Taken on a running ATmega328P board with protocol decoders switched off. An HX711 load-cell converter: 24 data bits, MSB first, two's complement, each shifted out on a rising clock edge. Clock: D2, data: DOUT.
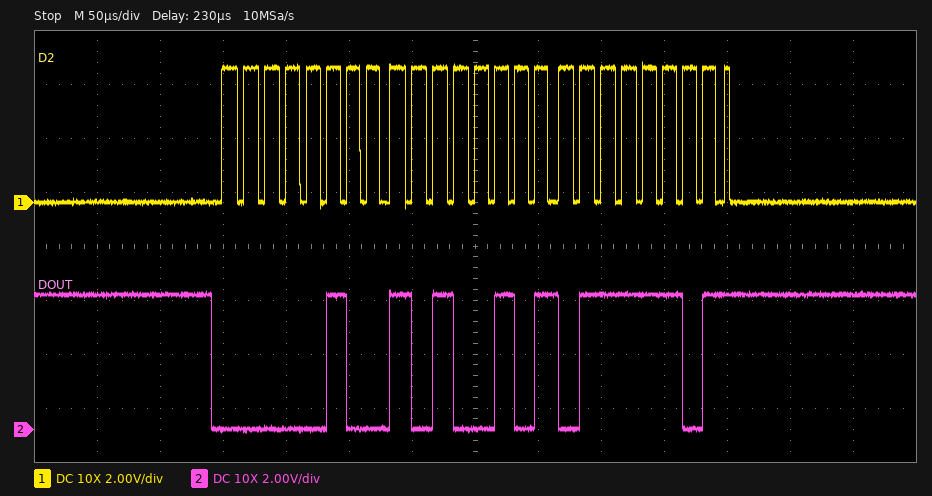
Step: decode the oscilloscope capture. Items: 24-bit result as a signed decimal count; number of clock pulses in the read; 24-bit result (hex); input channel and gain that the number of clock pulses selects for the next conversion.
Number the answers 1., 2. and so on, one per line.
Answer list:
1. 304509
2. 25
3. 0x04A57D
4. channel A, gain 128
